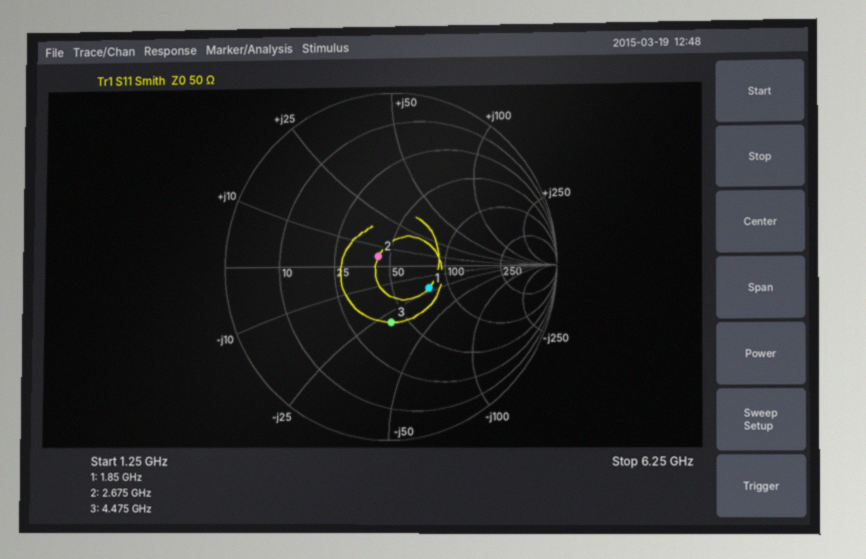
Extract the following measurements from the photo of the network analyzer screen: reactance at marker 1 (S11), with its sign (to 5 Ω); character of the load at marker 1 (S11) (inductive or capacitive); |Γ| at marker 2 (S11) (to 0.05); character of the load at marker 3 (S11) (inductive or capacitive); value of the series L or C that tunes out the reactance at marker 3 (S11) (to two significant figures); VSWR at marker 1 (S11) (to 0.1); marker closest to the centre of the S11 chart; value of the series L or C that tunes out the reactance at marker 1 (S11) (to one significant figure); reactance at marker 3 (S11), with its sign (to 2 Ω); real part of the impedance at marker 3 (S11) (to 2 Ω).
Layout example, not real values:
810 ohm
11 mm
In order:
-20 Ω
capacitive
0.10
capacitive
1.1 nH
1.7
marker 2
2 nH
-30 Ω
42 Ω
